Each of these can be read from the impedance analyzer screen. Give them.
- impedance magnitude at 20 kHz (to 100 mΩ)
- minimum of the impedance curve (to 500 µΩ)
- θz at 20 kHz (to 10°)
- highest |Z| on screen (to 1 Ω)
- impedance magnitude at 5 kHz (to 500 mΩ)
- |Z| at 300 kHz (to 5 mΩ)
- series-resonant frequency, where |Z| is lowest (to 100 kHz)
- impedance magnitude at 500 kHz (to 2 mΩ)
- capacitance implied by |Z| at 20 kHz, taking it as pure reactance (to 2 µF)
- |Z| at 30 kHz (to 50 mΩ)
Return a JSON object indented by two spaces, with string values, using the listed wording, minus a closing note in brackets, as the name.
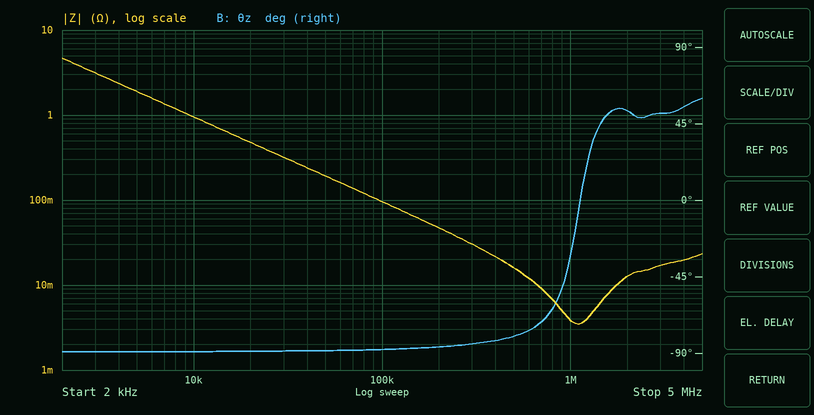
{
  "impedance magnitude at 20 kHz": "500 mΩ",
  "minimum of the impedance curve": "3.5 mΩ",
  "θz at 20 kHz": "-90°",
  "highest |Z| on screen": "5 Ω",
  "impedance magnitude at 5 kHz": "2.0 Ω",
  "|Z| at 300 kHz": "30 mΩ",
  "series-resonant frequency, where |Z| is lowest": "1.1 MHz",
  "impedance magnitude at 500 kHz": "16 mΩ",
  "capacitance implied by |Z| at 20 kHz, taking it as pure reactance": "16 µF",
  "|Z| at 30 kHz": "300 mΩ"
}
